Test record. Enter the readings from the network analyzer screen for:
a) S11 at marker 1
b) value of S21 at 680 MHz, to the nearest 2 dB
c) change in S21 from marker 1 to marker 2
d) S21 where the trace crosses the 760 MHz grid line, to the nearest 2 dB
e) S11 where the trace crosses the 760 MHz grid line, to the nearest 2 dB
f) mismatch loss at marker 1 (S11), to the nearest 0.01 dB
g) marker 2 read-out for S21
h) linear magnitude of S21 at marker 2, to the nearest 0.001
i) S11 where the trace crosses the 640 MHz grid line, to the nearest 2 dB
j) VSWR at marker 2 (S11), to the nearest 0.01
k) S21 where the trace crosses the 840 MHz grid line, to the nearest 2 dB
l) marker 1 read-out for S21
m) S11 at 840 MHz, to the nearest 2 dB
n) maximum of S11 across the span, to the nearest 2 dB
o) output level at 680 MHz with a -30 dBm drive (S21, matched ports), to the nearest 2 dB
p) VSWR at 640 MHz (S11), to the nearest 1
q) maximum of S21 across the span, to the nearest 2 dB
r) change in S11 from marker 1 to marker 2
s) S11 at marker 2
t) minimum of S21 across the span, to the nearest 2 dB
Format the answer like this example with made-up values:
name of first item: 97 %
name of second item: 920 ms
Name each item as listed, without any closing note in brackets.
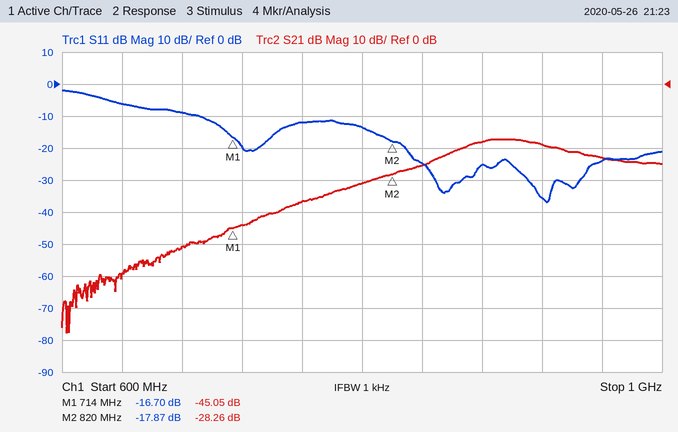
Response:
S11 at marker 1: -16.70 dB
value of S21 at 680 MHz, to the nearest 2 dB: -50 dB
change in S21 from marker 1 to marker 2: 16.79 dB
S21 where the trace crosses the 760 MHz grid line, to the nearest 2 dB: -36 dB
S11 where the trace crosses the 760 MHz grid line, to the nearest 2 dB: -12 dB
mismatch loss at marker 1 (S11), to the nearest 0.01 dB: 0.09 dB
marker 2 read-out for S21: -28.26 dB
linear magnitude of S21 at marker 2, to the nearest 0.001: 0.039
S11 where the trace crosses the 640 MHz grid line, to the nearest 2 dB: -6 dB
VSWR at marker 2 (S11), to the nearest 0.01: 1.29
S21 where the trace crosses the 840 MHz grid line, to the nearest 2 dB: -26 dB
marker 1 read-out for S21: -45.05 dB
S11 at 840 MHz, to the nearest 2 dB: -24 dB
maximum of S11 across the span, to the nearest 2 dB: -2 dB
output level at 680 MHz with a -30 dBm drive (S21, matched ports), to the nearest 2 dB: -80 dBm
VSWR at 640 MHz (S11), to the nearest 1: 3
maximum of S21 across the span, to the nearest 2 dB: -18 dB
change in S11 from marker 1 to marker 2: -1.17 dB
S11 at marker 2: -17.87 dB
minimum of S21 across the span, to the nearest 2 dB: -78 dB
